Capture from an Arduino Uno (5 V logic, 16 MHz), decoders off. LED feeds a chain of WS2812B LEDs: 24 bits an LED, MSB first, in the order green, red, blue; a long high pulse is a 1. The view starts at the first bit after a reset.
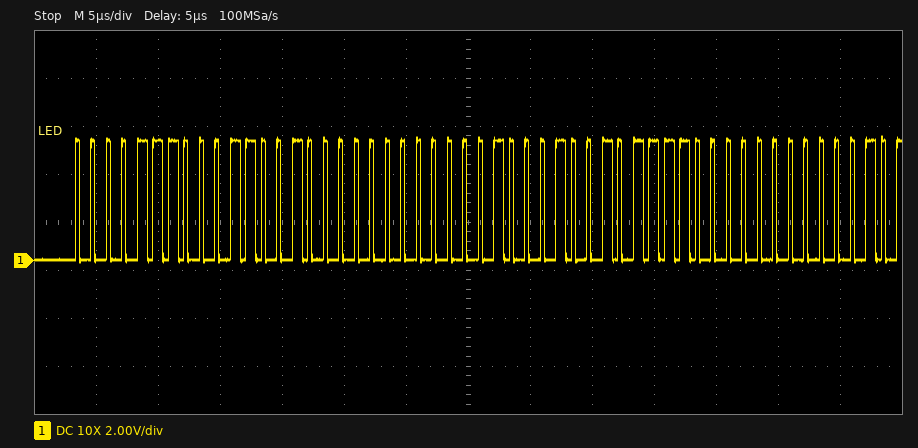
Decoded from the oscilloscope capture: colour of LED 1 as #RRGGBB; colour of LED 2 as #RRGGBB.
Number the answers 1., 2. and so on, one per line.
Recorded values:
1. #320E00
2. #2F1100
